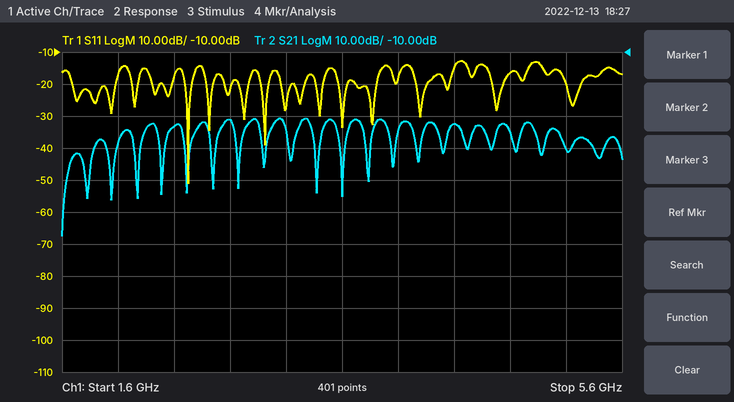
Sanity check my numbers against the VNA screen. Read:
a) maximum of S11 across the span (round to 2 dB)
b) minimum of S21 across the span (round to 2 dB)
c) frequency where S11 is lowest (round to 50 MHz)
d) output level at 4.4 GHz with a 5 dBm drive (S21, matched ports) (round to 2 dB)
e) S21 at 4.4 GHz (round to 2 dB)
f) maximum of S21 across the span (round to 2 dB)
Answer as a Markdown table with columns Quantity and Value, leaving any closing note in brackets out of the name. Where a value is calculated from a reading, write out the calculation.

| Quantity | Value |
|---|---|
| maximum of S11 across the span | -12 dB |
| minimum of S21 across the span | -68 dB |
| frequency where S11 is lowest | 2.50 GHz |
| output level at 4.4 GHz with a 5 dBm drive (S21, matched ports) | 5 dBm + (-32 dB) = -28 dBm |
| S21 at 4.4 GHz | -32 dB |
| maximum of S21 across the span | -30 dB |
